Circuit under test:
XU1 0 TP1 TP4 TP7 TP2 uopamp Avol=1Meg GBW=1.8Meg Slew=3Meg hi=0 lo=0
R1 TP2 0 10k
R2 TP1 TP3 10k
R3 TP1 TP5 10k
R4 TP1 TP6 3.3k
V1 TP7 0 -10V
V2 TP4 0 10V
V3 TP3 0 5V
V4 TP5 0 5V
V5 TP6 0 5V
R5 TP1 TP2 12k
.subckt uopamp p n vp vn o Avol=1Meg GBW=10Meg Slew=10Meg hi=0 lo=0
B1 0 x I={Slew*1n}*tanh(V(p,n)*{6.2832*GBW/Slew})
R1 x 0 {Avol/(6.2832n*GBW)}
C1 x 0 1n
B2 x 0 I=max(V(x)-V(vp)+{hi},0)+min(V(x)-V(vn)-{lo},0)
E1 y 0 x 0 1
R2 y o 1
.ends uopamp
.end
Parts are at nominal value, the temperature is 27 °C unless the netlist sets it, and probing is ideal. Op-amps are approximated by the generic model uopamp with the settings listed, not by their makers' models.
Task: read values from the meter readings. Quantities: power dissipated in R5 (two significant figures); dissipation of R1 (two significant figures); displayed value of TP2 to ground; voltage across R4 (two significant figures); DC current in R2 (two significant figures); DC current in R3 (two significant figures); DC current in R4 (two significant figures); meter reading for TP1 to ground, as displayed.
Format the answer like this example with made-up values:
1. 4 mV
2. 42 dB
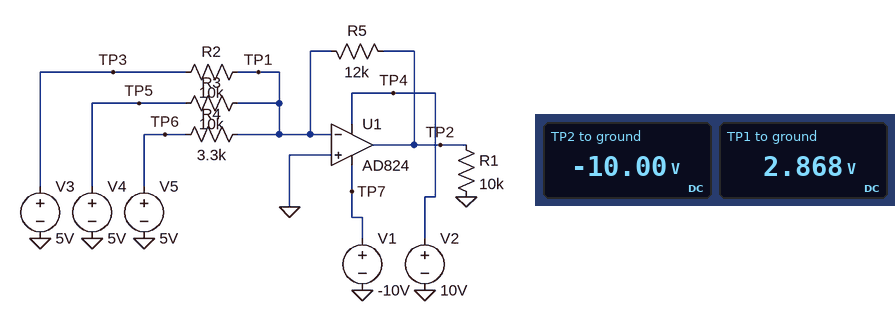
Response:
1. 14 mW
2. 10 mW
3. -10.00 V
4. 2.1 V
5. 210 µA
6. 210 µA
7. 650 µA
8. 2.868 V
